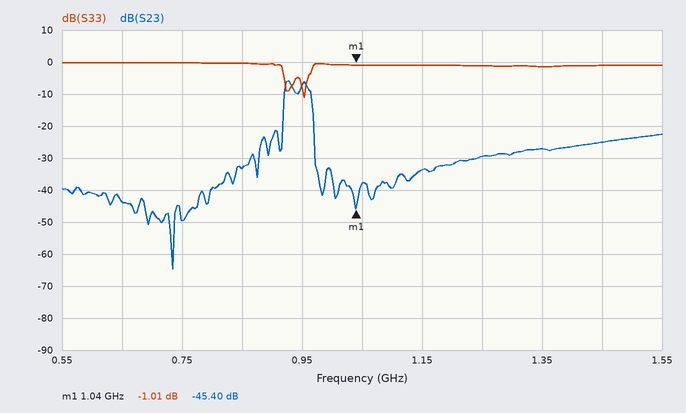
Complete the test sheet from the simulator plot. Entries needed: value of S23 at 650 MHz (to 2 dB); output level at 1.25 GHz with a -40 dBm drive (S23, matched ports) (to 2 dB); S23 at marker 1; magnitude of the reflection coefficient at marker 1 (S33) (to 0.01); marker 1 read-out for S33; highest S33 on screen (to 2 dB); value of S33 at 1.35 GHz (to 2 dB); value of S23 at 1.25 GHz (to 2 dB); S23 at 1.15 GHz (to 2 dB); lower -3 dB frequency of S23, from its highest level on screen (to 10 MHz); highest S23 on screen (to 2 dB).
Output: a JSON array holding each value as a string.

["-44 dB", "-70 dBm", "-45.40 dB", "0.89", "-1.01 dB", "0 dB", "-2 dB", "-30 dB", "-34 dB", "920 MHz", "-6 dB"]
